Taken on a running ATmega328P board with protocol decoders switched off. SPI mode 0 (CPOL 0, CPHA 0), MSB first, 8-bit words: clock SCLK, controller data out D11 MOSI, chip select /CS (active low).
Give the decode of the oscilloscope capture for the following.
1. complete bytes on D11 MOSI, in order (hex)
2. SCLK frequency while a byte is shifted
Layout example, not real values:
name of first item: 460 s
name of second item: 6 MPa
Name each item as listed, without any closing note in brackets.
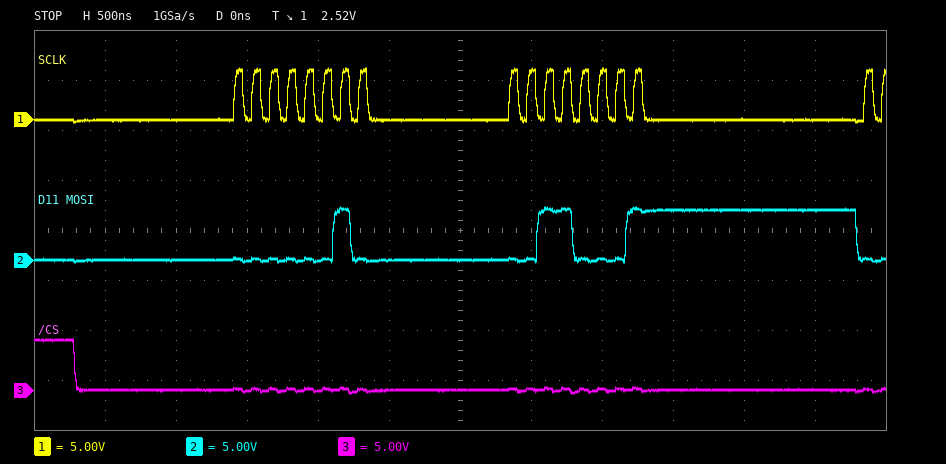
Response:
complete bytes on D11 MOSI, in order: 02 31
SCLK frequency while a byte is shifted: 8 MHz
